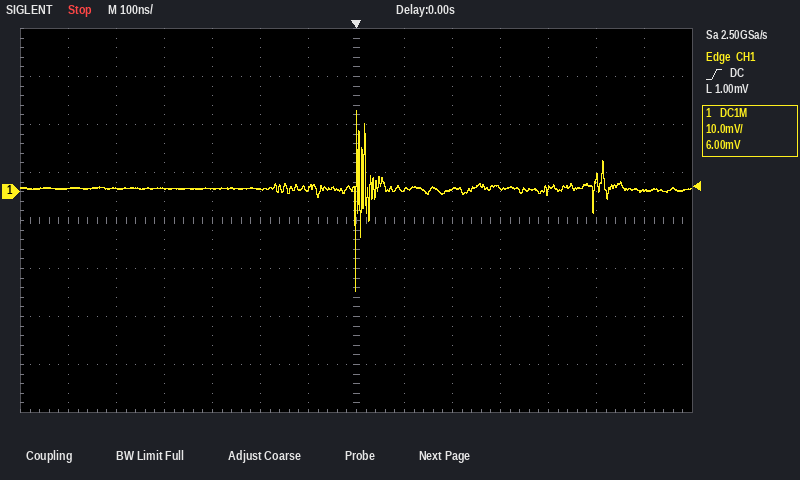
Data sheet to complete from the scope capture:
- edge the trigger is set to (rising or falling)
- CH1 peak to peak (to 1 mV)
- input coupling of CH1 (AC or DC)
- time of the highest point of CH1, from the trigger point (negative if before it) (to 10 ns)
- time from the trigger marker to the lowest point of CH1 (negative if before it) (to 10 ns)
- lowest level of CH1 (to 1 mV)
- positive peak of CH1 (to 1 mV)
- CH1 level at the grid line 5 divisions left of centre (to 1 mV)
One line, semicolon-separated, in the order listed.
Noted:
rising; 38 mV; DC; 0 ns; 0 ns; -21 mV; 17 mV; 1 mV
